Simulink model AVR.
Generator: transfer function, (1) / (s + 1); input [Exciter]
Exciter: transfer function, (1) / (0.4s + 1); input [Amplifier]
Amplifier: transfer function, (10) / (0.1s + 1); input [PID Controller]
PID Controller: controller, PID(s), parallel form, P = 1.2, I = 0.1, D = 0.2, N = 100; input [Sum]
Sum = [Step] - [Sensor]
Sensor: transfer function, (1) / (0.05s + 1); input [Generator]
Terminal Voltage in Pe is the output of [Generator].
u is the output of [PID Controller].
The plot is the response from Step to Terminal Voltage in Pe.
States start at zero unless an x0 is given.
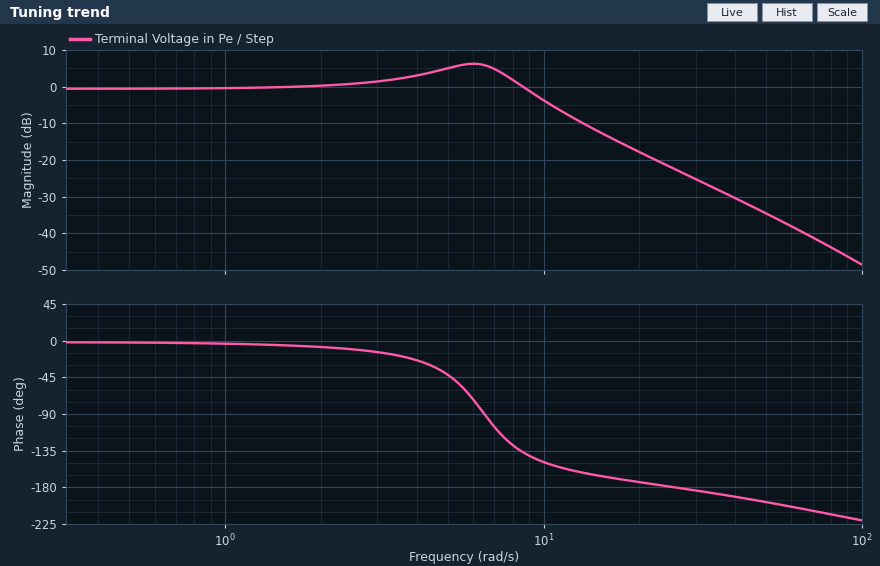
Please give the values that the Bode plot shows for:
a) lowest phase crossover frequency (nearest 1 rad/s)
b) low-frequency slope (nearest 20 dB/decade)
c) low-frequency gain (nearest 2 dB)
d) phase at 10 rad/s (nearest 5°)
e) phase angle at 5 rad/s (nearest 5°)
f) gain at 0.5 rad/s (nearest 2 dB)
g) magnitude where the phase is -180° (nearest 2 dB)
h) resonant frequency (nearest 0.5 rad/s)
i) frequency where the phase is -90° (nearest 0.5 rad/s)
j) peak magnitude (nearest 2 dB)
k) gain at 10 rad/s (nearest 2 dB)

26 rad/s
0 dB/decade
0 dB
-150°
-40°
0 dB
-22 dB
6.0 rad/s
6.5 rad/s
6 dB
-4 dB
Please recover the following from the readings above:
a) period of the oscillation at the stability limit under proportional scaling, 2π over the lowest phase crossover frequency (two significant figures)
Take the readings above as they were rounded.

0.24 s
